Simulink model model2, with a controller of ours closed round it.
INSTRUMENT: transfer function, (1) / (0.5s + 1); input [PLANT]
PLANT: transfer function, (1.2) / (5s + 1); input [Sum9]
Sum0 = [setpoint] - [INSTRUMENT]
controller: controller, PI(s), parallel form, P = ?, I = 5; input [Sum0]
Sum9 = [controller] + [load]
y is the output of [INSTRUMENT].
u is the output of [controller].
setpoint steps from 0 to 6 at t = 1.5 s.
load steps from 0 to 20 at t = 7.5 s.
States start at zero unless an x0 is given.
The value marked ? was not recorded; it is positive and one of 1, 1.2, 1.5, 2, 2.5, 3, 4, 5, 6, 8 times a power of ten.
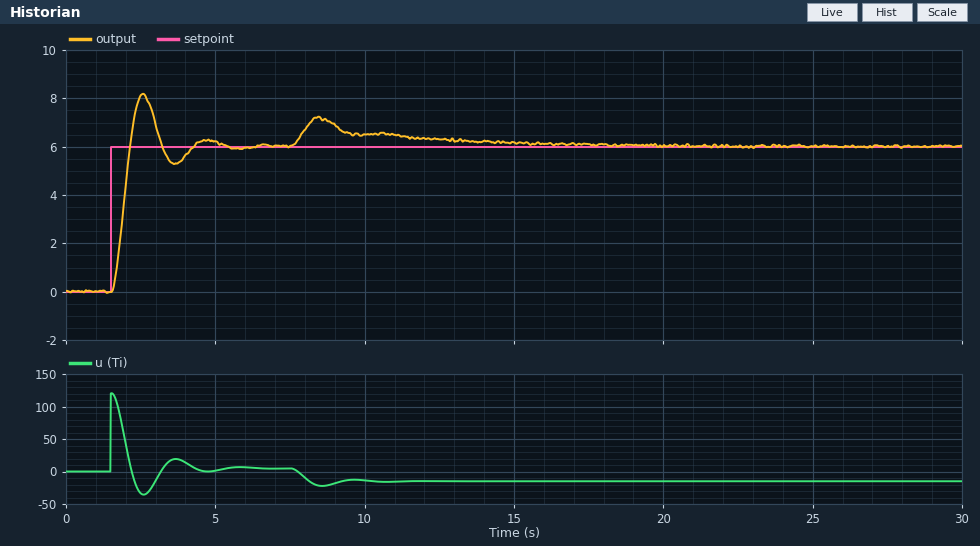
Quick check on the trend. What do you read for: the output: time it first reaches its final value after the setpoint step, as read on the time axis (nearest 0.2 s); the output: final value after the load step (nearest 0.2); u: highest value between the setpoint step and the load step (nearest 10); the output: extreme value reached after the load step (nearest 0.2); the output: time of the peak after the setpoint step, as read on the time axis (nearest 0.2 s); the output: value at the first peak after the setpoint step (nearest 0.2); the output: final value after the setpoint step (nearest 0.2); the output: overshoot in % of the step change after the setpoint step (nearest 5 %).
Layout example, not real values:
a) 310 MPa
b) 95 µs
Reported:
a) 2.2 s
b) 6.0
c) 120
d) 7.2
e) 2.6 s
f) 8.2
g) 6.0
h) 35 %
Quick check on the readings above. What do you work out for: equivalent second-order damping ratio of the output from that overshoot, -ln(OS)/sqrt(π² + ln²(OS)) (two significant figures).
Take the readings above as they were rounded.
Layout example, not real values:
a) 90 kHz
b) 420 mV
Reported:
a) 0.32
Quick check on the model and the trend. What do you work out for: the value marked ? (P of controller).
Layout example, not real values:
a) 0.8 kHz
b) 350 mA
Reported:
a) 20
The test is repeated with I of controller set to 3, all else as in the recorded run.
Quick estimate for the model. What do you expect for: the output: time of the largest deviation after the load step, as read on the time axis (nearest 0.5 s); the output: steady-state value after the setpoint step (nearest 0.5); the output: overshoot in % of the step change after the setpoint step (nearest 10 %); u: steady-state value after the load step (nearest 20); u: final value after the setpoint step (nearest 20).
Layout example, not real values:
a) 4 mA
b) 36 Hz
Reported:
a) 8.5 s
b) 6.0
c) 30 %
d) -20
e) 0
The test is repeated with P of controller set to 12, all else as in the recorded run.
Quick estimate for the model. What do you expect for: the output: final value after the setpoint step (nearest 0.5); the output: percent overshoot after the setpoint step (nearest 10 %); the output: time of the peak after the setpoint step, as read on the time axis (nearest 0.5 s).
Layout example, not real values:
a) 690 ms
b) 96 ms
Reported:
a) 6.0
b) 30 %
c) 3.0 s
